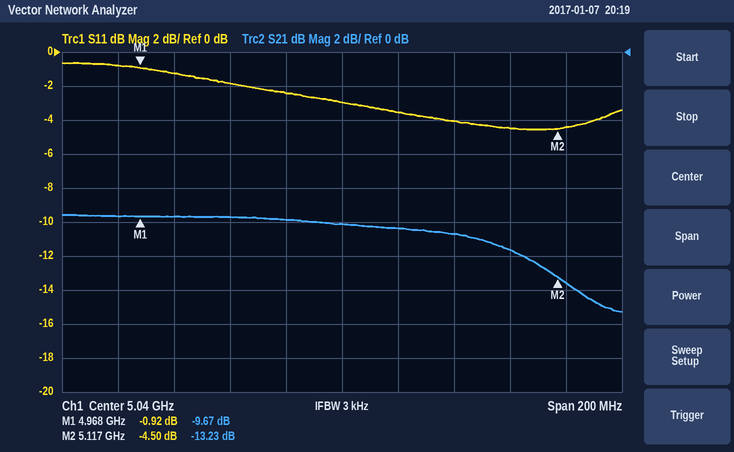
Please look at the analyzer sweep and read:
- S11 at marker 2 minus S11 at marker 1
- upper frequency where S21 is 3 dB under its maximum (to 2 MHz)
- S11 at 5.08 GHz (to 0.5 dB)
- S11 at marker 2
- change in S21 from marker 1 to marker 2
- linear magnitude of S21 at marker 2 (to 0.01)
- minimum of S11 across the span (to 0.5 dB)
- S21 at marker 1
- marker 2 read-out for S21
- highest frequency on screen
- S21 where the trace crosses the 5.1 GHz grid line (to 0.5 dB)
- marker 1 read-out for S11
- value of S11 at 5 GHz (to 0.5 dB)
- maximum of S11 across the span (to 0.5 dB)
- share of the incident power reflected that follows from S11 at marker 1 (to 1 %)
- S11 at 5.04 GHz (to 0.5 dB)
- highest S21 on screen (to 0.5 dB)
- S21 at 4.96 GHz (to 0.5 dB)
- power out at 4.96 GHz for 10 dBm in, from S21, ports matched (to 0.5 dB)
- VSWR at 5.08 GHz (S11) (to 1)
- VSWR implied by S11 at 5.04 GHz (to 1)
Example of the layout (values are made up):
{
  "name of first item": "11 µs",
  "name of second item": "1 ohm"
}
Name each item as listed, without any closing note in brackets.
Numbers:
{
  "S11 at marker 2 minus S11 at marker 1": "-3.58 dB",
  "upper frequency where S21 is 3 dB under its maximum": "5.110 GHz",
  "S11 at 5.08 GHz": "-4.0 dB",
  "S11 at marker 2": "-4.50 dB",
  "change in S21 from marker 1 to marker 2": "-3.56 dB",
  "linear magnitude of S21 at marker 2": "0.22",
  "minimum of S11 across the span": "-4.5 dB",
  "S21 at marker 1": "-9.67 dB",
  "marker 2 read-out for S21": "-13.23 dB",
  "highest frequency on screen": "5.14 GHz",
  "S21 where the trace crosses the 5.1 GHz grid line": "-11.5 dB",
  "marker 1 read-out for S11": "-0.92 dB",
  "value of S11 at 5 GHz": "-2.0 dB",
  "maximum of S11 across the span": "-0.5 dB",
  "share of the incident power reflected that follows from S11 at marker 1": "81 %",
  "S11 at 5.04 GHz": "-3.0 dB",
  "highest S21 on screen": "-9.5 dB",
  "S21 at 4.96 GHz": "-9.5 dB",
  "power out at 4.96 GHz for 10 dBm in, from S21, ports matched": "0.5 dBm",
  "VSWR at 5.08 GHz (S11)": "4",
  "VSWR implied by S11 at 5.04 GHz": "6"
}
